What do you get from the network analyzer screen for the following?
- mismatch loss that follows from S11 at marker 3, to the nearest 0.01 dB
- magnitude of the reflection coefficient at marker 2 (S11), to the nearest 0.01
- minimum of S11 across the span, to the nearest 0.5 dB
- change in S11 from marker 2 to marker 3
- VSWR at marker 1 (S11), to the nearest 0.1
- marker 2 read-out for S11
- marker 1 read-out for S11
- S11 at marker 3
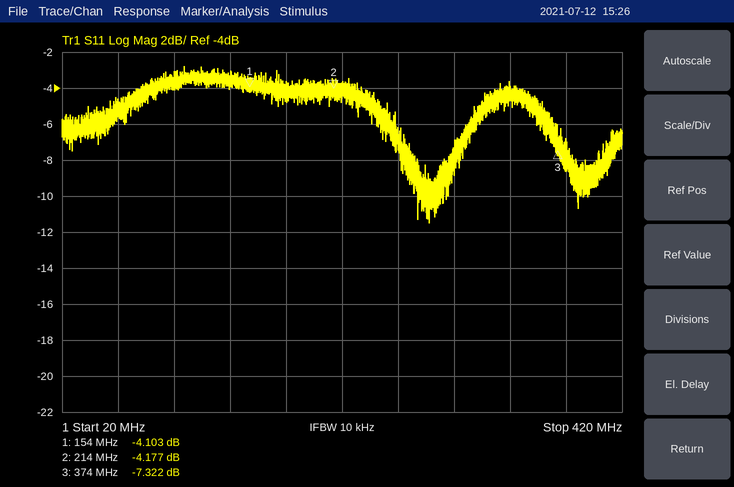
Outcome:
0.89 dB
0.62
-11.5 dB
-3.145 dB
4.3
-4.177 dB
-4.103 dB
-7.322 dB
